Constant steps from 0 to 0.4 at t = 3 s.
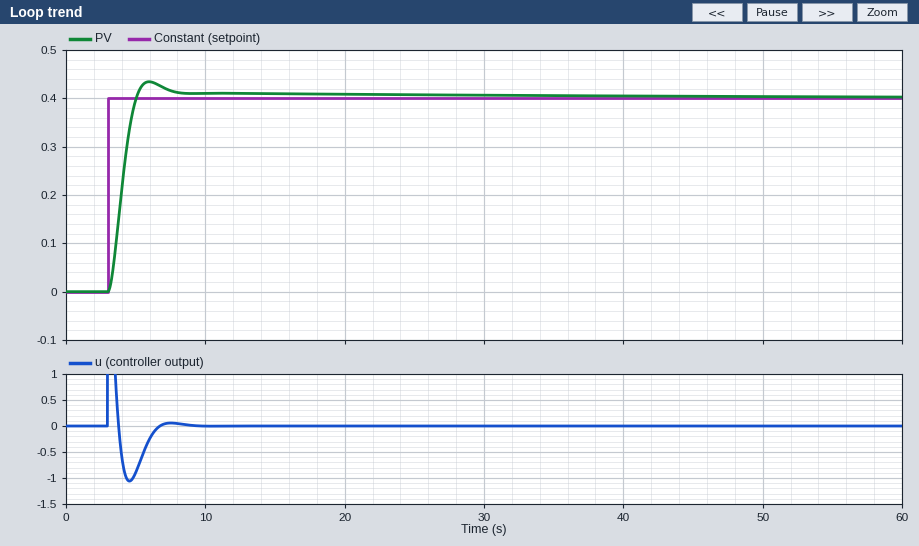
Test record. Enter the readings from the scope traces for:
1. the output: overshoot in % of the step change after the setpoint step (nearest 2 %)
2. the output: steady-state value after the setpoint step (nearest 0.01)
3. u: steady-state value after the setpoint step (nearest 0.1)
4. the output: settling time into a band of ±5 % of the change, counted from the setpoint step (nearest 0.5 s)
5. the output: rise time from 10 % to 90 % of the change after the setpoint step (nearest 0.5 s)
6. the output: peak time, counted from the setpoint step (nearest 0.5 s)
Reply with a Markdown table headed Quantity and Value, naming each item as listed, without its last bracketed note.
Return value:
| Quantity | Value |
|---|---|
| the output: overshoot in % of the step change after the setpoint step | 8 % |
| the output: steady-state value after the setpoint step | 0.40 |
| u: steady-state value after the setpoint step | 0.0 |
| the output: settling time into a band of ±5 % of the change, counted from the setpoint step | 4.0 s |
| the output: rise time from 10 % to 90 % of the change after the setpoint step | 1.5 s |
| the output: peak time, counted from the setpoint step | 3.0 s |
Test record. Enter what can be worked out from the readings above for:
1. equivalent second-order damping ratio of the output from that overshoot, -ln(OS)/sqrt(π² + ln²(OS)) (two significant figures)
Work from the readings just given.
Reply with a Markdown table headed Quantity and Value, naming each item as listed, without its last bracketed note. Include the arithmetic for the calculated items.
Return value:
| Quantity | Value |
|---|---|
| equivalent second-order damping ratio of the output from that overshoot, -ln(OS)/sqrt(π² + ln²(OS)) | ln(0.08) = -2.526; 2.526 / sqrt(9.870 + 6.379) = 0.63 |
